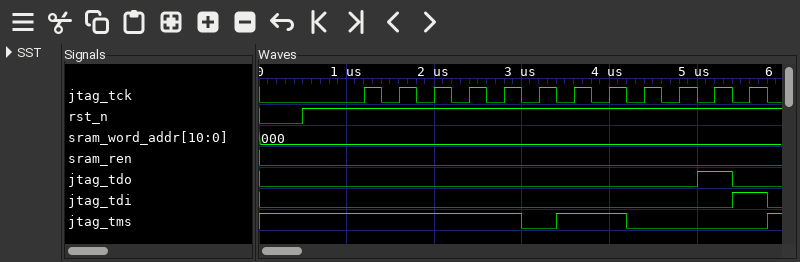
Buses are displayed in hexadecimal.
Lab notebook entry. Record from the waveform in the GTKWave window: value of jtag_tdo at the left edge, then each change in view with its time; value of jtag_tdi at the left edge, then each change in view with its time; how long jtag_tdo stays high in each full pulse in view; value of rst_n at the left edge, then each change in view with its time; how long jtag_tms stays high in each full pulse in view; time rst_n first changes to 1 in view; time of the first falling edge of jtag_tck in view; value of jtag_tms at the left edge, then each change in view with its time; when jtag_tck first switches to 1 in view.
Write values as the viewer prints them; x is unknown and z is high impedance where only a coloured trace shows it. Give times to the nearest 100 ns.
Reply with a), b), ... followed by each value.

a) 0, 1 at 5000 ns, 0 at 5400 ns
b) 0, 1 at 5400 ns, 0 at 5800 ns
c) 400 ns
d) 0, 1 at 500 ns
e) 800 ns
f) 500 ns
g) 1400 ns
h) 1, 0 at 3000 ns, 1 at 3400 ns, 0 at 4200 ns, 1 at 5800 ns
i) 1200 ns
